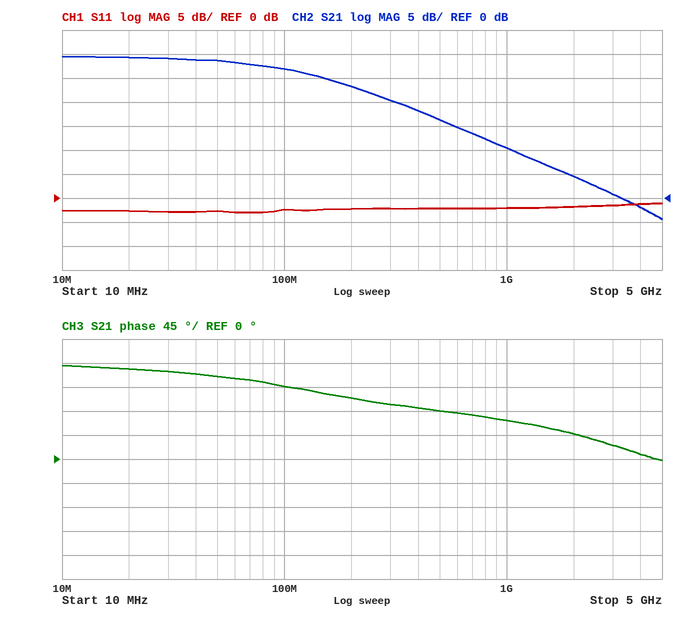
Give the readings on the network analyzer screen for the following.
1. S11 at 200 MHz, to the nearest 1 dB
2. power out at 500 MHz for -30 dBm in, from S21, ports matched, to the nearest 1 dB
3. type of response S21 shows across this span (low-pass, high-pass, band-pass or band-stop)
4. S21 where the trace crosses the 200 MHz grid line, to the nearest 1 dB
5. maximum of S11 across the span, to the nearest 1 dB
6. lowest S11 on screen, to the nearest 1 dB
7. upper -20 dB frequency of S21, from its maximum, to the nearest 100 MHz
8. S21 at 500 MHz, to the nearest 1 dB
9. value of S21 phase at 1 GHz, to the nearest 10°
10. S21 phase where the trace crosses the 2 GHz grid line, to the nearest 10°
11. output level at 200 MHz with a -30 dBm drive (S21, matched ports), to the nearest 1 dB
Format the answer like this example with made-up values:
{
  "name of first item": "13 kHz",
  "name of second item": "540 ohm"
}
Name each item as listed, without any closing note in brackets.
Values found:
{
  "S11 at 200 MHz, to the nearest 1 dB": "-2 dB",
  "power out at 500 MHz for -30 dBm in, from S21, ports matched, to the nearest 1 dB": "-14 dBm",
  "type of response S21 shows across this span": "low-pass",
  "S21 where the trace crosses the 200 MHz grid line, to the nearest 1 dB": "23 dB",
  "maximum of S11 across the span, to the nearest 1 dB": "-1 dB",
  "lowest S11 on screen, to the nearest 1 dB": "-3 dB",
  "upper -20 dB frequency of S21, from its maximum, to the nearest 100 MHz": "1.1 GHz",
  "S21 at 500 MHz, to the nearest 1 dB": "16 dB",
  "value of S21 phase at 1 GHz, to the nearest 10°": "70°",
  "S21 phase where the trace crosses the 2 GHz grid line, to the nearest 10°": "50°",
  "output level at 200 MHz with a -30 dBm drive (S21, matched ports), to the nearest 1 dB": "-7 dBm"
}
